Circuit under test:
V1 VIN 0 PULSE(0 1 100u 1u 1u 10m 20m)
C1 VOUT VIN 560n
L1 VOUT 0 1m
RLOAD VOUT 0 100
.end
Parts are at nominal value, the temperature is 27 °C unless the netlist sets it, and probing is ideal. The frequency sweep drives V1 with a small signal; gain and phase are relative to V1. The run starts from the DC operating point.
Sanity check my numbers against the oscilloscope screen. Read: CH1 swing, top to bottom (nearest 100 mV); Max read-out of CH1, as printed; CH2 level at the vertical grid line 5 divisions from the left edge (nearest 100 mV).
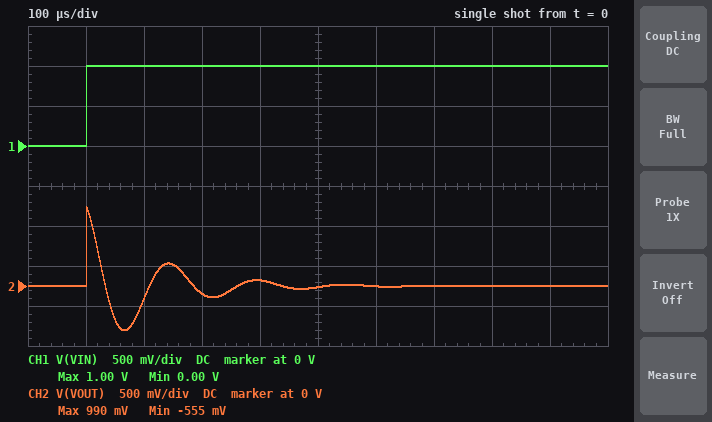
1.0 V
1.00 V
0 V
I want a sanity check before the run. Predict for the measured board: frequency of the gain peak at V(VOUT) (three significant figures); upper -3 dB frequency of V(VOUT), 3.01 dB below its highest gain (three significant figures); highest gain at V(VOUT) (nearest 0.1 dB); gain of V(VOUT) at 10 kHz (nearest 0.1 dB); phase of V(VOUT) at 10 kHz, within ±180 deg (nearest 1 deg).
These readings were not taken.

7.05 kHz
9.53 kHz
7.7 dB
4.2 dB
27 deg
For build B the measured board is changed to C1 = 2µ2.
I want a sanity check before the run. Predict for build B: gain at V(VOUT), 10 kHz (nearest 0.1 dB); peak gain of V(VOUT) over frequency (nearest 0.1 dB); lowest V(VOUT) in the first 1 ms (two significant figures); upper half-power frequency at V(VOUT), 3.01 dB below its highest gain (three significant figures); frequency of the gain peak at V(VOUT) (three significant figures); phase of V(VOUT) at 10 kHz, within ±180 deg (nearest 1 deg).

1.0 dB
13.5 dB
-730 mV
3.88 kHz
3.43 kHz
5 deg
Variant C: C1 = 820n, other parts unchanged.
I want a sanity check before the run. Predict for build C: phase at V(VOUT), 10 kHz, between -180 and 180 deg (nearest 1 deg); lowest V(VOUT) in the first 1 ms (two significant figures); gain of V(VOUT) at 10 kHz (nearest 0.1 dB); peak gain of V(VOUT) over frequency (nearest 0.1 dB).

16 deg
-610 mV
2.9 dB
9.3 dB
